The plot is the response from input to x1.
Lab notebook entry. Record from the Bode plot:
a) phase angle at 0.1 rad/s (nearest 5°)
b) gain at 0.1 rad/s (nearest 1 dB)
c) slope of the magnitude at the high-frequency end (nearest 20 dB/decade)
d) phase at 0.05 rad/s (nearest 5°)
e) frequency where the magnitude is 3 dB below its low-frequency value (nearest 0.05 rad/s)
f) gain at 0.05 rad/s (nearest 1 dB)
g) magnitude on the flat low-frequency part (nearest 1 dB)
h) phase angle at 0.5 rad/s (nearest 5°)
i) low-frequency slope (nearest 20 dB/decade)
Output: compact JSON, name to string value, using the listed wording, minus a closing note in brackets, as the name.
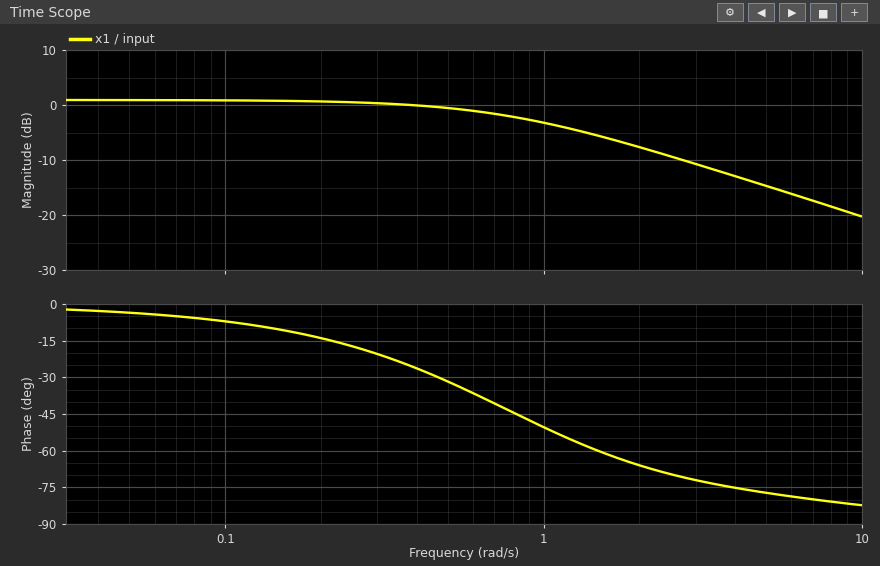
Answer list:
{"phase angle at 0.1 rad/s": "-5°", "gain at 0.1 rad/s": "1 dB", "slope of the magnitude at the high-frequency end": "-20 dB/decade", "phase at 0.05 rad/s": "-5°", "frequency where the magnitude is 3 dB below its low-frequency value": "0.80 rad/s", "gain at 0.05 rad/s": "1 dB", "magnitude on the flat low-frequency part": "1 dB", "phase angle at 0.5 rad/s": "-30°", "low-frequency slope": "0 dB/decade"}
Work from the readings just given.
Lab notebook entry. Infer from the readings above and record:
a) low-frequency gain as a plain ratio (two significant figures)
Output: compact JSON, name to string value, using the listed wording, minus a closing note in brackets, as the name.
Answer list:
{"low-frequency gain as a plain ratio": "1.1"}
